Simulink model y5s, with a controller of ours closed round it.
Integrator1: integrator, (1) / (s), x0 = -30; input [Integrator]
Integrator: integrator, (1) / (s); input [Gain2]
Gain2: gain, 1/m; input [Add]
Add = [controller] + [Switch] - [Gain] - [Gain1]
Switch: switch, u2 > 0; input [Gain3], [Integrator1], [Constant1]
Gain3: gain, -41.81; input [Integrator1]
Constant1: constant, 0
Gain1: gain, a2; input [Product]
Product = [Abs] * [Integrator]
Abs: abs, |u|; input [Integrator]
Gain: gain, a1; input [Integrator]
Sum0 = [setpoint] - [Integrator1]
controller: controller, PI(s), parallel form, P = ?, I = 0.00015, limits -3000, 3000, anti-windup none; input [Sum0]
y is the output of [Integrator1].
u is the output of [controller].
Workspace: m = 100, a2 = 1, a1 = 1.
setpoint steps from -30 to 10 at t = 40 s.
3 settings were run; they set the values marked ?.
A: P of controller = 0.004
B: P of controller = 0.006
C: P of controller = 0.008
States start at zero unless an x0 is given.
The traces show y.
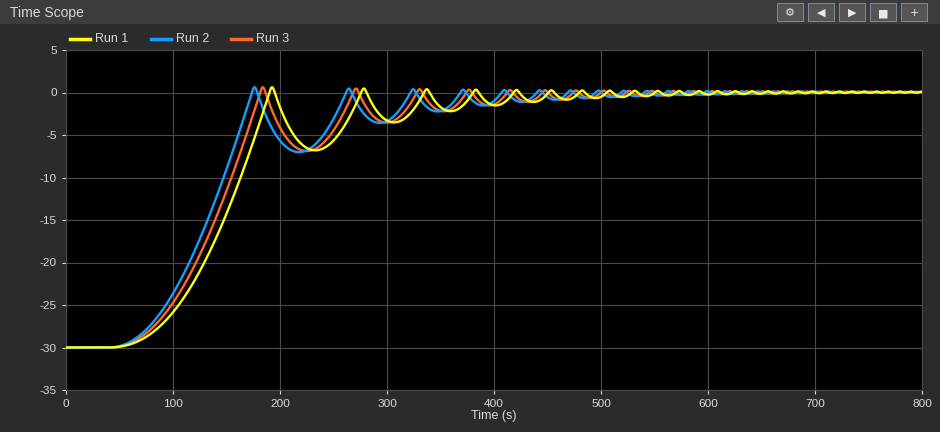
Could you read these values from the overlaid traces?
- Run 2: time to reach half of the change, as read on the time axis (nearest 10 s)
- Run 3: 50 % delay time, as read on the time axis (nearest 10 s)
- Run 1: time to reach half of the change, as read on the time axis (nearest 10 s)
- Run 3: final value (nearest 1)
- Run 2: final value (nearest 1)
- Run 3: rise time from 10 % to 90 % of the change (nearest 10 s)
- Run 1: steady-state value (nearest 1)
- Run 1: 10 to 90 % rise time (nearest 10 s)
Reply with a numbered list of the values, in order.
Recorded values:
1. 130 s
2. 140 s
3. 150 s
4. 0
5. 0
6. 90 s
7. 0
8. 90 s
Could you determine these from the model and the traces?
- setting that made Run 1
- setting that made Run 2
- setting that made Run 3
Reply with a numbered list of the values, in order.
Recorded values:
1. A
2. C
3. B
